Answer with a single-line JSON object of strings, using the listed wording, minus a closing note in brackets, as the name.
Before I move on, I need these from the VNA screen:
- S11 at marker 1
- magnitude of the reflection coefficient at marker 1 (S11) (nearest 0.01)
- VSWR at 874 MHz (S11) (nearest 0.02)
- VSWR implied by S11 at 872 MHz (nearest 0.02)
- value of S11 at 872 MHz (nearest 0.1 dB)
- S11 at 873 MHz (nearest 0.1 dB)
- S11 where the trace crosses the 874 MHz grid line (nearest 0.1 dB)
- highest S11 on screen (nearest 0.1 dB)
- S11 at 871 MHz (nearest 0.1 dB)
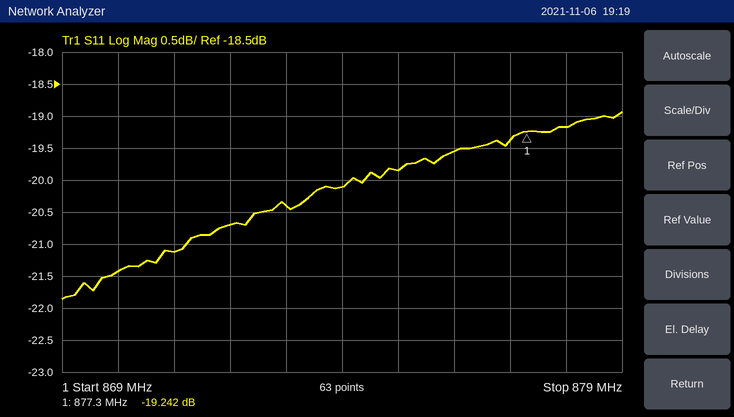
{"S11 at marker 1": "-19.242 dB", "magnitude of the reflection coefficient at marker 1 (S11)": "0.11", "VSWR at 874 MHz (S11)": "1.22", "VSWR implied by S11 at 872 MHz": "1.20", "value of S11 at 872 MHz": "-20.7 dB", "S11 at 873 MHz": "-20.4 dB", "S11 where the trace crosses the 874 MHz grid line": "-20.1 dB", "highest S11 on screen": "-18.9 dB", "S11 at 871 MHz": "-21.1 dB"}
